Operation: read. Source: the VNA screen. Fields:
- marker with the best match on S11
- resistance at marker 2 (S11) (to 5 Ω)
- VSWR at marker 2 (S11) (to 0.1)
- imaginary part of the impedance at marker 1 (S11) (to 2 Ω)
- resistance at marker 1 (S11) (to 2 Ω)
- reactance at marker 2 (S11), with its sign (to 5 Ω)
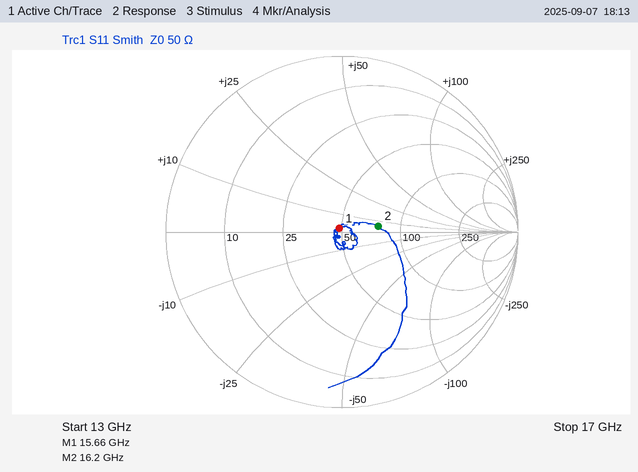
marker 1
75 Ω
1.5
+2 Ω
48 Ω
+5 Ω
